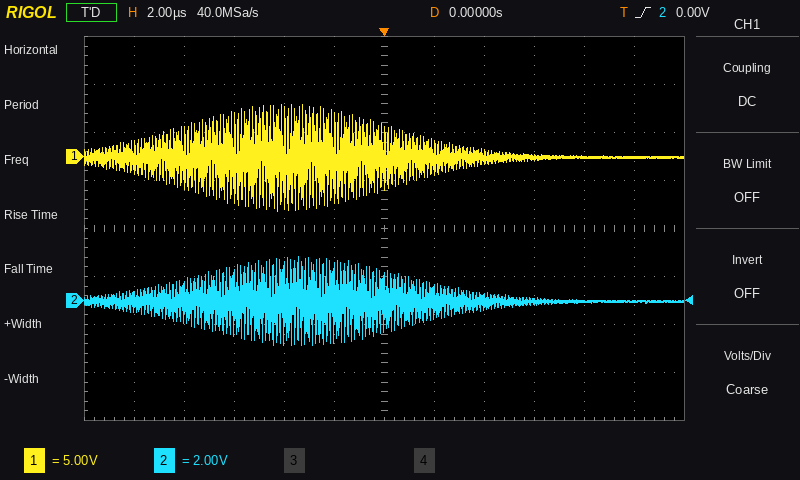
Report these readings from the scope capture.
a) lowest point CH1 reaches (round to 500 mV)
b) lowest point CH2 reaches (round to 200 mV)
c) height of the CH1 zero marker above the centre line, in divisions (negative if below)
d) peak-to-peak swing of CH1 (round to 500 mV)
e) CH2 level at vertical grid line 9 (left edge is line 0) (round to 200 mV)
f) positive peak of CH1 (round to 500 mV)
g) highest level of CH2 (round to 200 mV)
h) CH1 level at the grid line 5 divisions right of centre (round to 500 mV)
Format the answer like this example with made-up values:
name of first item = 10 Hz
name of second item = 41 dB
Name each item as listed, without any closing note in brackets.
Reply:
lowest point CH1 reaches = -5.5 V
lowest point CH2 reaches = -1.8 V
height of the CH1 zero marker above the centre line, in divisions = +1.5 div
peak-to-peak swing of CH1 = 11.0 V
CH2 level at vertical grid line 9 (left edge is line 0) = 0.0 V
positive peak of CH1 = 5.5 V
highest level of CH2 = 1.8 V
CH1 level at the grid line 5 divisions right of centre = 0.0 V
